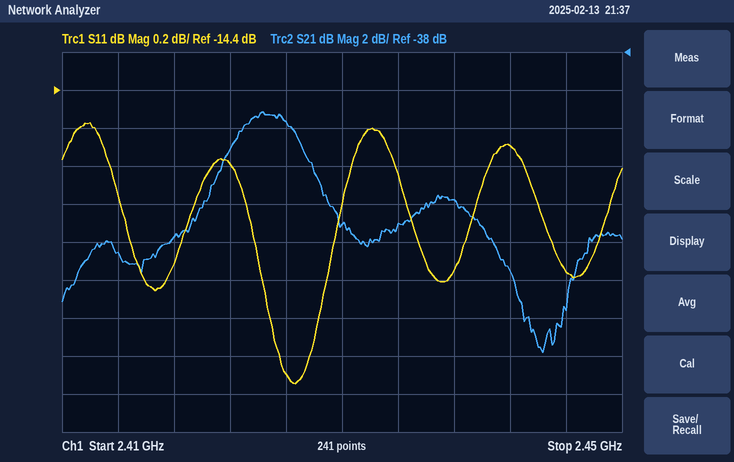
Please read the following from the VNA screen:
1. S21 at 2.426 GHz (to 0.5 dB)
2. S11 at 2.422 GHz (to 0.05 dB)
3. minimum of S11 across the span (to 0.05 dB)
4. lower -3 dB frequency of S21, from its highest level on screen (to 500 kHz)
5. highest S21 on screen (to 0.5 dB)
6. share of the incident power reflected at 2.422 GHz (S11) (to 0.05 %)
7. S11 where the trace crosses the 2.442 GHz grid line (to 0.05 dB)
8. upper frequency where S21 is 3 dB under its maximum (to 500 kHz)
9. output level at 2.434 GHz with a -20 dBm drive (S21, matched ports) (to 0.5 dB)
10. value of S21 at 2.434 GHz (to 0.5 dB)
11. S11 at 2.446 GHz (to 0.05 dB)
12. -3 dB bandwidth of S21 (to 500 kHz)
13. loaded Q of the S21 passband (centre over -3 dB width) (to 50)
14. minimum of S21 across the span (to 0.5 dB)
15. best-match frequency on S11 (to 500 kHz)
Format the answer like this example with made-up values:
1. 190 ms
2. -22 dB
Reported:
1. -41.5 dB
2. -14.80 dB
3. -15.95 dB
4. 2.4215 GHz
5. -41.0 dB
6. 3.30 %
7. -14.70 dB
8. 2.4280 GHz
9. -67.0 dBm
10. -47.0 dB
11. -15.35 dB
12. 6.5 MHz
13. 350
14. -54.0 dB
15. 2.4265 GHz
